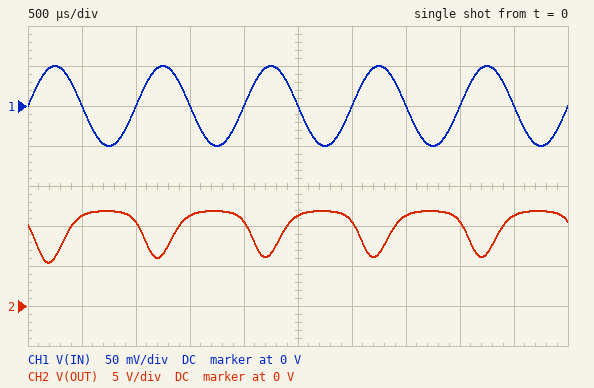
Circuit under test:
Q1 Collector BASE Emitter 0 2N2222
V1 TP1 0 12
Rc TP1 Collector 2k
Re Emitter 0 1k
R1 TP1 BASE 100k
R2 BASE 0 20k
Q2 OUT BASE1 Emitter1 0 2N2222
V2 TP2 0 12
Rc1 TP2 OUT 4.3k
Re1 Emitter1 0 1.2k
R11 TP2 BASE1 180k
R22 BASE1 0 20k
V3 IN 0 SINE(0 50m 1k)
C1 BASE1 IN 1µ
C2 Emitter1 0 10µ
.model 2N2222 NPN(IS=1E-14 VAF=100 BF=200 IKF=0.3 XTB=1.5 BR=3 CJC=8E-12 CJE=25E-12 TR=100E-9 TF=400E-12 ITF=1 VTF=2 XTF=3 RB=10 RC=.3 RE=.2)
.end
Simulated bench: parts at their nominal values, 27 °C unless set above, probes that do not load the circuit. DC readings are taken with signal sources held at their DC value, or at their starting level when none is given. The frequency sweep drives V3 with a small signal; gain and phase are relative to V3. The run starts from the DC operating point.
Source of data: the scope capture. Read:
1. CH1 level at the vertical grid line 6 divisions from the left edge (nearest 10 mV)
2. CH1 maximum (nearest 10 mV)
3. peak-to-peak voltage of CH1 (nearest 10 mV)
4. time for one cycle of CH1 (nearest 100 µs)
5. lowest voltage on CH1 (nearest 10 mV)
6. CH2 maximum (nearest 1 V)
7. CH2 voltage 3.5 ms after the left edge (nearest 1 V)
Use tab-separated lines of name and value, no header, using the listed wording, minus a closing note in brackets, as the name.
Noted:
CH1 level at the vertical grid line 6 divisions from the left edge	0 V
CH1 maximum	50 mV
peak-to-peak voltage of CH1	100 mV
time for one cycle of CH1	1.0 ms
lowest voltage on CH1	-50 mV
CH2 maximum	12 V
CH2 voltage 3.5 ms after the left edge	11 V
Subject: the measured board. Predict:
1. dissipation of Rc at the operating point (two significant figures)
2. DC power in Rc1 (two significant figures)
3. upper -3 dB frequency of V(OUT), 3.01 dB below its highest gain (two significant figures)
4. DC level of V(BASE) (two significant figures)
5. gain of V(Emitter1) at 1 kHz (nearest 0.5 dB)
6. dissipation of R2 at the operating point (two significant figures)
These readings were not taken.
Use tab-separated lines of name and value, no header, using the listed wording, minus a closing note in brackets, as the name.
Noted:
dissipation of Rc at the operating point	3.1 mW
DC power in Rc1	840 µW
upper -3 dB frequency of V(OUT), 3.01 dB below its highest gain	9.3 MHz
DC level of V(BASE)	1.9 V
gain of V(Emitter1) at 1 kHz	-12.0 dB
dissipation of R2 at the operating point	180 µW
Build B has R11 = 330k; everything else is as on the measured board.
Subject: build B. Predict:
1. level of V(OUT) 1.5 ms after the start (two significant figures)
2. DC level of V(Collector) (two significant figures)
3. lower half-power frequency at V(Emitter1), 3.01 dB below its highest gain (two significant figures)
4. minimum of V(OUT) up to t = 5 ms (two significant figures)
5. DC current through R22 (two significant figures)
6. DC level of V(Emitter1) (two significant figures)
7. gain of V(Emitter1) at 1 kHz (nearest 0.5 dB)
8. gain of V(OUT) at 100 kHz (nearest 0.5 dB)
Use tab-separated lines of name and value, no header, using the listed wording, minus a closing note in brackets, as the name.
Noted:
level of V(OUT) 1.5 ms after the start	12 V
DC level of V(Collector)	9.5 V
lower half-power frequency at V(Emitter1), 3.01 dB below its highest gain	6.9 Hz
minimum of V(OUT) up to t = 5 ms	10 V
DC current through R22	34 µA
DC level of V(Emitter1)	93 mV
gain of V(Emitter1) at 1 kHz	-26.5 dB
gain of V(OUT) at 100 kHz	22.0 dB
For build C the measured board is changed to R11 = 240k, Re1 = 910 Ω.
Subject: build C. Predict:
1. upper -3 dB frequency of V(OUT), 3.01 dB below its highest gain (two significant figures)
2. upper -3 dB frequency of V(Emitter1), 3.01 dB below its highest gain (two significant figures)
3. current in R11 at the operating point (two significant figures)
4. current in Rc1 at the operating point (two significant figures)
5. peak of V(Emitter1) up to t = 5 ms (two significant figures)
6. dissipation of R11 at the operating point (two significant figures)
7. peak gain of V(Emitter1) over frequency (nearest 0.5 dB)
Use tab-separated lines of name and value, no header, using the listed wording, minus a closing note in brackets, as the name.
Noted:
upper -3 dB frequency of V(OUT), 3.01 dB below its highest gain	10 MHz
upper -3 dB frequency of V(Emitter1), 3.01 dB below its highest gain	230 Hz
current in R11 at the operating point	46 µA
current in Rc1 at the operating point	300 µA
peak of V(Emitter1) up to t = 5 ms	300 mV
dissipation of R11 at the operating point	510 µW
peak gain of V(Emitter1) over frequency	-1.5 dB
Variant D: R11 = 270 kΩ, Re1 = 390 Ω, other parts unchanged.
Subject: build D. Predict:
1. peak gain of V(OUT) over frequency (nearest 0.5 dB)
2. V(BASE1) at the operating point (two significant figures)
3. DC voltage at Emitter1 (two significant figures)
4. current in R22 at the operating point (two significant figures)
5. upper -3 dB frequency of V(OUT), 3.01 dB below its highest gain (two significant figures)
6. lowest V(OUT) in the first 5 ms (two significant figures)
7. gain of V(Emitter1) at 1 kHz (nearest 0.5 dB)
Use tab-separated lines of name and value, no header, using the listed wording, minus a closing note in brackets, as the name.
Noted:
peak gain of V(OUT) over frequency	36.5 dB
V(BASE1) at the operating point	790 mV
DC voltage at Emitter1	160 mV
current in R22 at the operating point	40 µA
upper -3 dB frequency of V(OUT), 3.01 dB below its highest gain	9.5 MHz
lowest V(OUT) in the first 5 ms	5.7 V
gain of V(Emitter1) at 1 kHz	-12.5 dB
